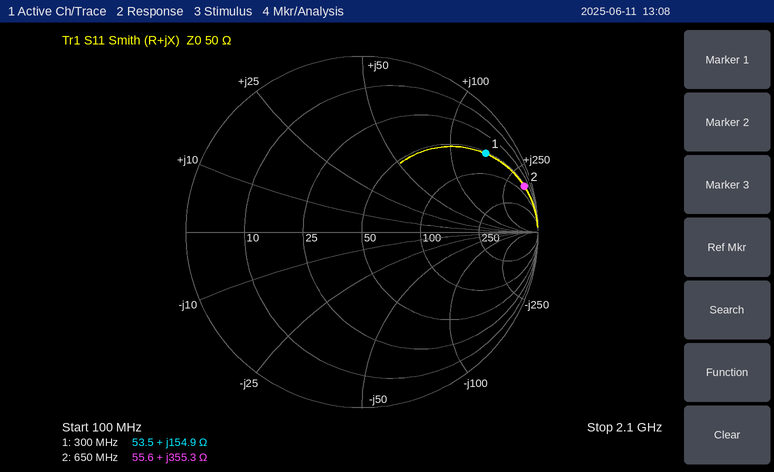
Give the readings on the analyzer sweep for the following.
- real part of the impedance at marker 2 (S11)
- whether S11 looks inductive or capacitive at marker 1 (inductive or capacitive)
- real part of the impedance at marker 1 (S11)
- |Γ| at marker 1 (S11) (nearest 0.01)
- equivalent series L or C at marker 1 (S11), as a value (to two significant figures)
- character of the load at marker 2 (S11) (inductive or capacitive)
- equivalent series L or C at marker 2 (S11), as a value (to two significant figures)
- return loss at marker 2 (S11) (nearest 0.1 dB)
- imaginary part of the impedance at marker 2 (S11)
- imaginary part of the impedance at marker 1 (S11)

55.6 Ω
inductive
53.5 Ω
0.83
82 nH
inductive
87 nH
0.4 dB
+355.3 Ω
+154.9 Ω
